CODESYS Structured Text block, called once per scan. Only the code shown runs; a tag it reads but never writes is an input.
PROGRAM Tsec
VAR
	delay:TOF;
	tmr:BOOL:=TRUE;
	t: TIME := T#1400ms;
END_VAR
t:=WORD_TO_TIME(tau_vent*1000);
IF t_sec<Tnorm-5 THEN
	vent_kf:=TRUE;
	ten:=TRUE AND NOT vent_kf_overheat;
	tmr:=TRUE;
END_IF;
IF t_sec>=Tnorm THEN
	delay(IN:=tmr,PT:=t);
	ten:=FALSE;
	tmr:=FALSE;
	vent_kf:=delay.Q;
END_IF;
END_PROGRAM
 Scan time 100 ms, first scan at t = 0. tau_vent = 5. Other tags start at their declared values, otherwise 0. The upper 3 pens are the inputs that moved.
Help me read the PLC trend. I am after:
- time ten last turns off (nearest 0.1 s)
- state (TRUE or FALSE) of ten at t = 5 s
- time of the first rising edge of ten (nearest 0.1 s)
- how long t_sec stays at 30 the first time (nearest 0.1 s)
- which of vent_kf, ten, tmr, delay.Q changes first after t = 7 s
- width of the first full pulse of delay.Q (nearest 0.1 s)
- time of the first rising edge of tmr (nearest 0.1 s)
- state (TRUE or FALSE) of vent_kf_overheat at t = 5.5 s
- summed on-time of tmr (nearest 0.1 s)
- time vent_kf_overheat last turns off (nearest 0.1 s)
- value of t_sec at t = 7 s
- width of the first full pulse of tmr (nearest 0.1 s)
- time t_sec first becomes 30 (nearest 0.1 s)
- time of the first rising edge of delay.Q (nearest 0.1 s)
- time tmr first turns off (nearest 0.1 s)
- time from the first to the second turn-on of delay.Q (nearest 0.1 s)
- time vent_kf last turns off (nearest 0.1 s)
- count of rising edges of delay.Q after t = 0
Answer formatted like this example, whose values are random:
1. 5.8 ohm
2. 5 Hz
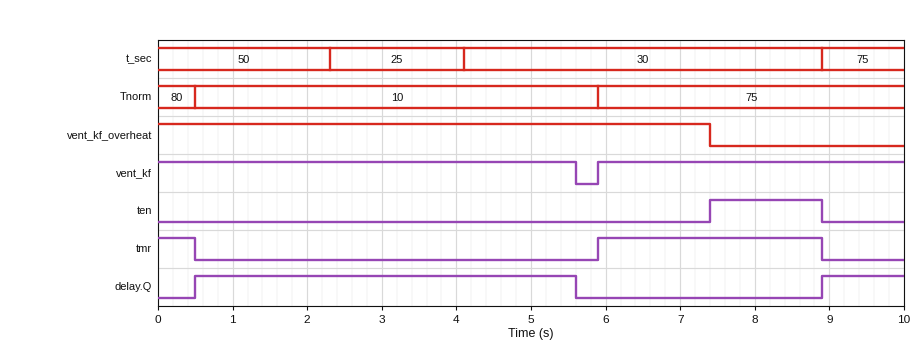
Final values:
1. 8.9 s
2. FALSE
3. 7.4 s
4. 4.8 s
5. ten
6. 5.1 s
7. 5.9 s
8. TRUE
9. 3.5 s
10. 7.4 s
11. 30
12. 3.0 s
13. 4.1 s
14. 0.5 s
15. 0.5 s
16. 8.4 s
17. 5.6 s
18. 2
